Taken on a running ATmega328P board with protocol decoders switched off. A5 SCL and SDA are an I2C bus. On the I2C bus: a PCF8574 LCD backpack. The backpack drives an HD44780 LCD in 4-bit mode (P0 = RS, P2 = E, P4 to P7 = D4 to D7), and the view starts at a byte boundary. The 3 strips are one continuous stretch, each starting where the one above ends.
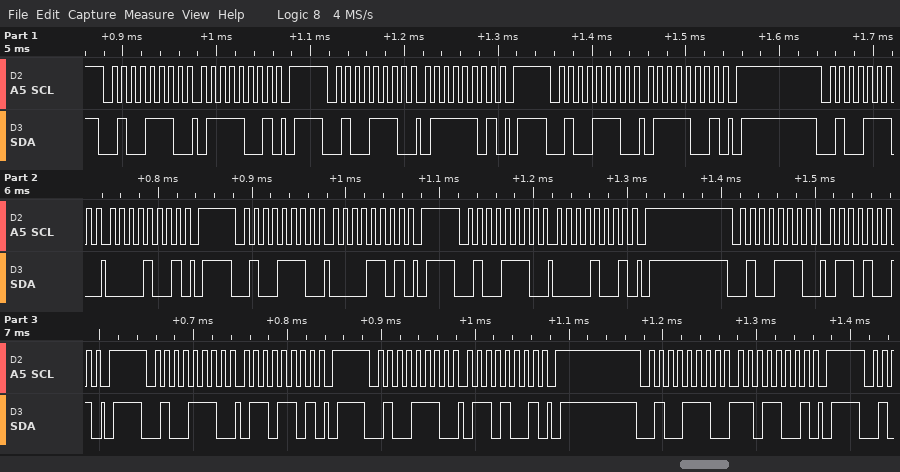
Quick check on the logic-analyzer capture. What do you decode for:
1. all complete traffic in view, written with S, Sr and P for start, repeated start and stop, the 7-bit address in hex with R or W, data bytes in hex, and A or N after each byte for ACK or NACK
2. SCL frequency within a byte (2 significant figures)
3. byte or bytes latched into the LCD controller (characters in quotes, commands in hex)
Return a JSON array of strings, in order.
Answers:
["S 27W A 79 A P S 27W A 7D A P S 27W A 79 A P S 27W A 09 A P S 27W A 0D A P S 27W A 09 A P S 27W A 69 A P S 27W A 6D A P S 27W A 69 A P S 27W A D9 A P", "100 kHz", "'p'"]
